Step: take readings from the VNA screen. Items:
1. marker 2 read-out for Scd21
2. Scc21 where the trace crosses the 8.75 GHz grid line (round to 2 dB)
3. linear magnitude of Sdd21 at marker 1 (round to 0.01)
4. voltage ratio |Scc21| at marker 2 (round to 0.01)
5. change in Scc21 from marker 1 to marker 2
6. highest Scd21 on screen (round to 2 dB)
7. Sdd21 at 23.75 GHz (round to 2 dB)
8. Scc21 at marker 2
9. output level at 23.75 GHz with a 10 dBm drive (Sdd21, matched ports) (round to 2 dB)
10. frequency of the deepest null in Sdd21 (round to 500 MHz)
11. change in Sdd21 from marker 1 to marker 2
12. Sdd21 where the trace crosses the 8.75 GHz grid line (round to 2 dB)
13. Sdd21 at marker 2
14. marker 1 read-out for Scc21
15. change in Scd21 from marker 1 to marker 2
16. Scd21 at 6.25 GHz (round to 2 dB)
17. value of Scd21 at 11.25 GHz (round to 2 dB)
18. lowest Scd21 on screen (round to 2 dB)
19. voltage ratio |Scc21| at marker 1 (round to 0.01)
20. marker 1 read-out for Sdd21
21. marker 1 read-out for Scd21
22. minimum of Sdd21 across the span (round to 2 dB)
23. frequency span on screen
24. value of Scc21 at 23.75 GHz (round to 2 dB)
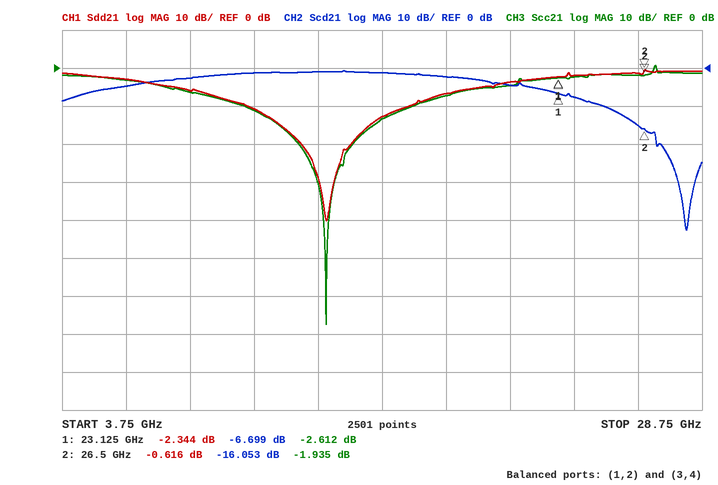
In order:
-16.053 dB
-6 dB
0.76
0.80
0.677 dB
0 dB
-2 dB
-1.935 dB
8 dBm
14.0 GHz
1.728 dB
-6 dB
-0.616 dB
-2.612 dB
-9.354 dB
-4 dB
-2 dB
-42 dB
0.74
-2.344 dB
-6.699 dB
-40 dB
25 GHz
-2 dB
